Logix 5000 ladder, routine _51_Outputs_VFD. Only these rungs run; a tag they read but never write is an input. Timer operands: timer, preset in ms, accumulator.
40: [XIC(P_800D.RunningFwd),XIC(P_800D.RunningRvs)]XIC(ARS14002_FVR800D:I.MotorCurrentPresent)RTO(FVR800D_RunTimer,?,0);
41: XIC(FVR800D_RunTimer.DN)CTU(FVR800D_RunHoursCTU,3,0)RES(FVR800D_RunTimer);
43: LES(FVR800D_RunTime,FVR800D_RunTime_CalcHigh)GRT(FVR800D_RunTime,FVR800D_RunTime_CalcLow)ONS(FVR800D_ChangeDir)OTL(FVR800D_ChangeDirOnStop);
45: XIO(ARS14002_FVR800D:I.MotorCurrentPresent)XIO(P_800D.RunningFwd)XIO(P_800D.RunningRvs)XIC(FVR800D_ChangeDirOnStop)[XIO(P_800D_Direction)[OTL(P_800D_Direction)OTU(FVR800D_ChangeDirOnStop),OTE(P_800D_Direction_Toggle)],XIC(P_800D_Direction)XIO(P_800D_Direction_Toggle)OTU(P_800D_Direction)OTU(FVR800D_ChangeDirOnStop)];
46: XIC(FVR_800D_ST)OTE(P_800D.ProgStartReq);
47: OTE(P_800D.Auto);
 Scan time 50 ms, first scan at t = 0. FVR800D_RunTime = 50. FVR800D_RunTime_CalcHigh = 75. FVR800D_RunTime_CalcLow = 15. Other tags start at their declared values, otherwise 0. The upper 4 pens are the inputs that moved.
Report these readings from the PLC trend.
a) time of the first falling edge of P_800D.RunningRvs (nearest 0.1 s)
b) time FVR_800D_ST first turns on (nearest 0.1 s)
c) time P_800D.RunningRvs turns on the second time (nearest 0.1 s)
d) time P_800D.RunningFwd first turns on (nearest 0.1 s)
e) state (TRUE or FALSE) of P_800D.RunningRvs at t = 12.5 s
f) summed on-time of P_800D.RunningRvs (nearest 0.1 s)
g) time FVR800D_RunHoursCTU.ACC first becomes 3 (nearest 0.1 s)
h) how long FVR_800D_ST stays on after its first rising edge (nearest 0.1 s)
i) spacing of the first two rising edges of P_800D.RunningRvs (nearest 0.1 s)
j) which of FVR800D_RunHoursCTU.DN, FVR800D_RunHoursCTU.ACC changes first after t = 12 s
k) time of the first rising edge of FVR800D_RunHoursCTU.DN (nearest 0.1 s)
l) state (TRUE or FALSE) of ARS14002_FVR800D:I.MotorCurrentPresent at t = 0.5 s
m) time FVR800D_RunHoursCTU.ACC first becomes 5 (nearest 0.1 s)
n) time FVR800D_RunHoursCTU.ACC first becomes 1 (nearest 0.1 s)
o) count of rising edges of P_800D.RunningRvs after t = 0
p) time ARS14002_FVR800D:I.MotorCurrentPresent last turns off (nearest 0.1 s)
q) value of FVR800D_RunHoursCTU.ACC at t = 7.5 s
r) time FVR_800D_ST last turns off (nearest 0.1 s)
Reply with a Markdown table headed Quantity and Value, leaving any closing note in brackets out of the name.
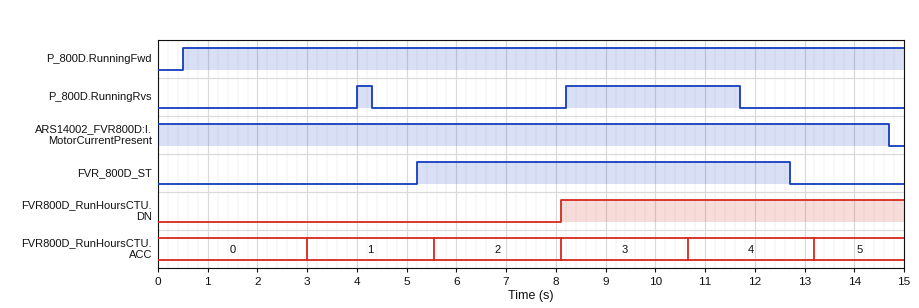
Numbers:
| Quantity | Value |
|---|---|
| time of the first falling edge of P_800D.RunningRvs | 4.3 s |
| time FVR_800D_ST first turns on | 5.2 s |
| time P_800D.RunningRvs turns on the second time | 8.2 s |
| time P_800D.RunningFwd first turns on | 0.5 s |
| state (TRUE or FALSE) of P_800D.RunningRvs at t = 12.5 s | FALSE |
| summed on-time of P_800D.RunningRvs | 3.8 s |
| time FVR800D_RunHoursCTU.ACC first becomes 3 | 8.1 s |
| how long FVR_800D_ST stays on after its first rising edge | 7.5 s |
| spacing of the first two rising edges of P_800D.RunningRvs | 4.2 s |
| which of FVR800D_RunHoursCTU.DN, FVR800D_RunHoursCTU.ACC changes first after t = 12 s | FVR800D_RunHoursCTU.ACC |
| time of the first rising edge of FVR800D_RunHoursCTU.DN | 8.1 s |
| state (TRUE or FALSE) of ARS14002_FVR800D:I.MotorCurrentPresent at t = 0.5 s | TRUE |
| time FVR800D_RunHoursCTU.ACC first becomes 5 | 13.2 s |
| time FVR800D_RunHoursCTU.ACC first becomes 1 | 3.0 s |
| count of rising edges of P_800D.RunningRvs after t = 0 | 2 |
| time ARS14002_FVR800D:I.MotorCurrentPresent last turns off | 14.7 s |
| value of FVR800D_RunHoursCTU.ACC at t = 7.5 s | 2 |
| time FVR_800D_ST last turns off | 12.7 s |
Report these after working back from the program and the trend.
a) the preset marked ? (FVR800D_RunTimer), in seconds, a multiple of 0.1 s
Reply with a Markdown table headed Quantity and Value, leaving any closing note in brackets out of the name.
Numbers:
| Quantity | Value |
|---|---|
| the preset marked ? (FVR800D_RunTimer), in seconds, a multiple of 0.1 s | 2.5 s |
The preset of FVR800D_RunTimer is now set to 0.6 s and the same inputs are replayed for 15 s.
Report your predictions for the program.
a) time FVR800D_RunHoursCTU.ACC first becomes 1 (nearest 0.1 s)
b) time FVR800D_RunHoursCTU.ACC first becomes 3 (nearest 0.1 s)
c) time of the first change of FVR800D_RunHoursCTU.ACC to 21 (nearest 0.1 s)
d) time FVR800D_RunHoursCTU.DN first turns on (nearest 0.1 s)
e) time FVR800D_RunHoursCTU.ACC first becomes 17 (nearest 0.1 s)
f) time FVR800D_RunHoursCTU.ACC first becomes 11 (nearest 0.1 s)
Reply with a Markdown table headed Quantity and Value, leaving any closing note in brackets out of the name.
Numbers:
| Quantity | Value |
|---|---|
| time FVR800D_RunHoursCTU.ACC first becomes 1 | 1.1 s |
| time FVR800D_RunHoursCTU.ACC first becomes 3 | 2.4 s |
| time of the first change of FVR800D_RunHoursCTU.ACC to 21 | 14.1 s |
| time FVR800D_RunHoursCTU.DN first turns on | 2.4 s |
| time FVR800D_RunHoursCTU.ACC first becomes 17 | 11.5 s |
| time FVR800D_RunHoursCTU.ACC first becomes 11 | 7.6 s |
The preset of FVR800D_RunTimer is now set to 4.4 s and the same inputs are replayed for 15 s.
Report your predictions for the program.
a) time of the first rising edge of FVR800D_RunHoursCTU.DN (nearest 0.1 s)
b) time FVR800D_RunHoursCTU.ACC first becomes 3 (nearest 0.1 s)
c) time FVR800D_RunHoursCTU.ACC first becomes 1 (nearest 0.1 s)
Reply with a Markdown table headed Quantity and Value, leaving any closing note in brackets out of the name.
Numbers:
| Quantity | Value |
|---|---|
| time of the first rising edge of FVR800D_RunHoursCTU.DN | 13.8 s |
| time FVR800D_RunHoursCTU.ACC first becomes 3 | 13.8 s |
| time FVR800D_RunHoursCTU.ACC first becomes 1 | 4.9 s |
